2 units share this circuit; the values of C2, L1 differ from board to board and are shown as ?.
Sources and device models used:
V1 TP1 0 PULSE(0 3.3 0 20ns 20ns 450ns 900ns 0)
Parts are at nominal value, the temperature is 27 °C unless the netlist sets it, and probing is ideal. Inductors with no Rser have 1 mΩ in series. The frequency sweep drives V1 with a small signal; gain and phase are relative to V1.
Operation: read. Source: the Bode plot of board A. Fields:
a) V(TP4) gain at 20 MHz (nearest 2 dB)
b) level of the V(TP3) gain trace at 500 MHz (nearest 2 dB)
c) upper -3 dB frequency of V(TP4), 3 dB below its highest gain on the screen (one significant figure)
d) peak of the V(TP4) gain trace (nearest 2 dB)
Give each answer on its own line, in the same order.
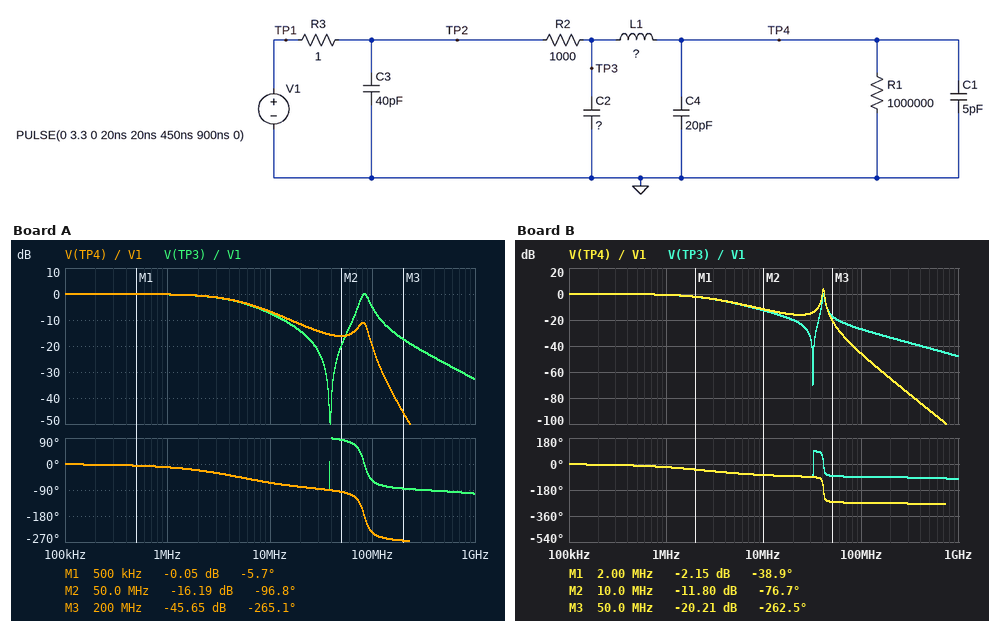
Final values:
-12 dB
-26 dB
5 MHz
0 dB
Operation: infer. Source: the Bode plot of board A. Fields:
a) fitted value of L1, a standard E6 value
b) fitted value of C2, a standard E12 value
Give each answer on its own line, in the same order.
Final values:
680 nH
6.8 pF
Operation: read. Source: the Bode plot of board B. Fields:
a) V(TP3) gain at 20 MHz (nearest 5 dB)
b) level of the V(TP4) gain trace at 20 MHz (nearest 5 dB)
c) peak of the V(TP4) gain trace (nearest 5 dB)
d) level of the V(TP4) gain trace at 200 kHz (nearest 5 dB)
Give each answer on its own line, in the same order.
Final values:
-20 dB
-15 dB
5 dB
0 dB
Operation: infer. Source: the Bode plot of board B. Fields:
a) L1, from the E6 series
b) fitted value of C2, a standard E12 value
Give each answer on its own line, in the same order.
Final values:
1 µH
39 pF
